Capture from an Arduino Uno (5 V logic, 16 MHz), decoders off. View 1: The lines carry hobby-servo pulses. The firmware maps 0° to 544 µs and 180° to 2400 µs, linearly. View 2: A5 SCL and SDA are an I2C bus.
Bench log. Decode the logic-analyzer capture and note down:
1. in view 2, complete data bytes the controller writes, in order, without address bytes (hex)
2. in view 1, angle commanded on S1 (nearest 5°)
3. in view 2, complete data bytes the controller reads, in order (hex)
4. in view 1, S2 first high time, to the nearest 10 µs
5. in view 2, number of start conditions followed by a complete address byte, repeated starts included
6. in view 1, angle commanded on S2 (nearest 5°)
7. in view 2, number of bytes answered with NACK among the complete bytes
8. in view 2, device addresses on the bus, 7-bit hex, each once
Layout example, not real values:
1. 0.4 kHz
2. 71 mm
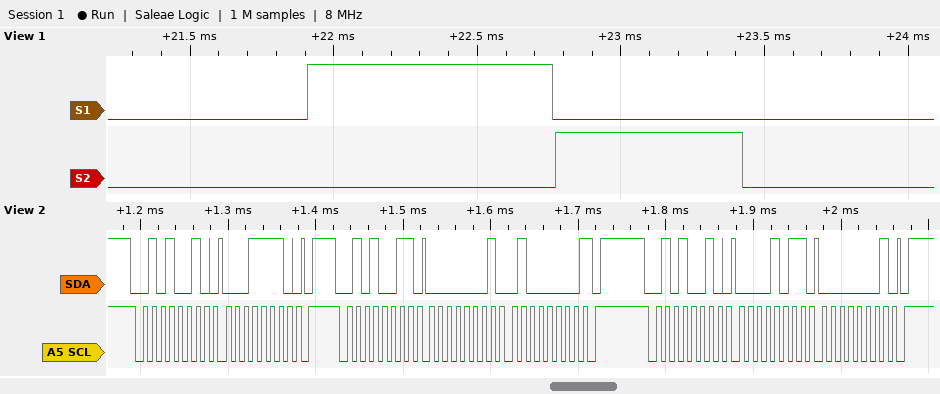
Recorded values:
1. 1E 0B 01
2. 30°
3. 01 40
4. 650 µs
5. 3
6. 10°
7. 1
8. 0x29
